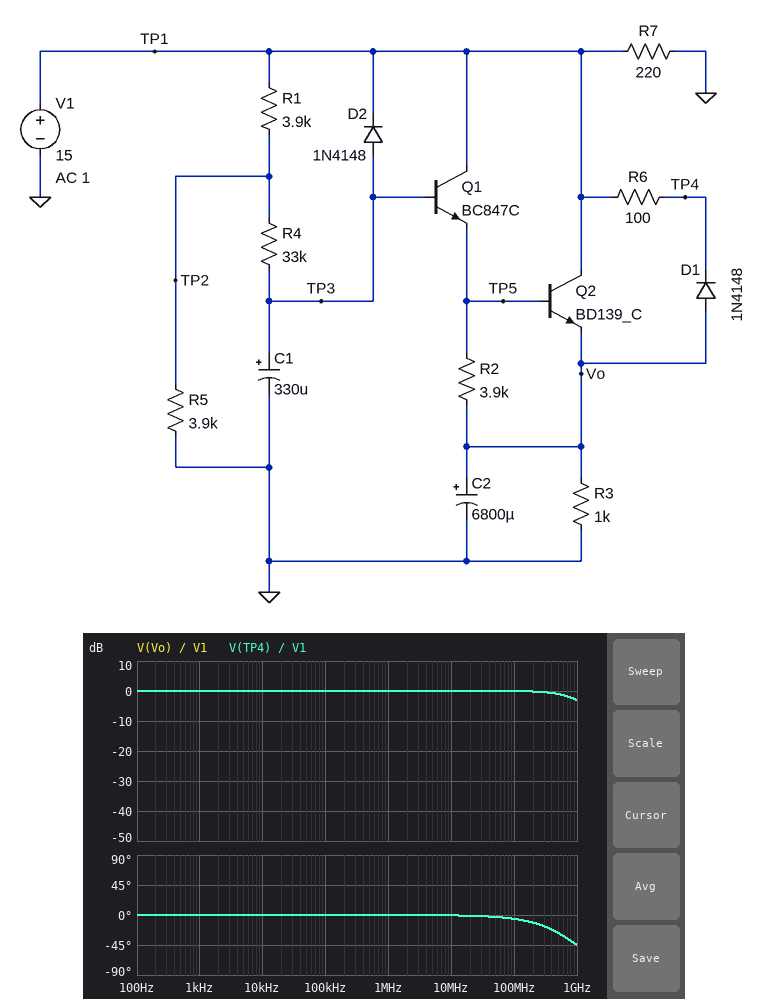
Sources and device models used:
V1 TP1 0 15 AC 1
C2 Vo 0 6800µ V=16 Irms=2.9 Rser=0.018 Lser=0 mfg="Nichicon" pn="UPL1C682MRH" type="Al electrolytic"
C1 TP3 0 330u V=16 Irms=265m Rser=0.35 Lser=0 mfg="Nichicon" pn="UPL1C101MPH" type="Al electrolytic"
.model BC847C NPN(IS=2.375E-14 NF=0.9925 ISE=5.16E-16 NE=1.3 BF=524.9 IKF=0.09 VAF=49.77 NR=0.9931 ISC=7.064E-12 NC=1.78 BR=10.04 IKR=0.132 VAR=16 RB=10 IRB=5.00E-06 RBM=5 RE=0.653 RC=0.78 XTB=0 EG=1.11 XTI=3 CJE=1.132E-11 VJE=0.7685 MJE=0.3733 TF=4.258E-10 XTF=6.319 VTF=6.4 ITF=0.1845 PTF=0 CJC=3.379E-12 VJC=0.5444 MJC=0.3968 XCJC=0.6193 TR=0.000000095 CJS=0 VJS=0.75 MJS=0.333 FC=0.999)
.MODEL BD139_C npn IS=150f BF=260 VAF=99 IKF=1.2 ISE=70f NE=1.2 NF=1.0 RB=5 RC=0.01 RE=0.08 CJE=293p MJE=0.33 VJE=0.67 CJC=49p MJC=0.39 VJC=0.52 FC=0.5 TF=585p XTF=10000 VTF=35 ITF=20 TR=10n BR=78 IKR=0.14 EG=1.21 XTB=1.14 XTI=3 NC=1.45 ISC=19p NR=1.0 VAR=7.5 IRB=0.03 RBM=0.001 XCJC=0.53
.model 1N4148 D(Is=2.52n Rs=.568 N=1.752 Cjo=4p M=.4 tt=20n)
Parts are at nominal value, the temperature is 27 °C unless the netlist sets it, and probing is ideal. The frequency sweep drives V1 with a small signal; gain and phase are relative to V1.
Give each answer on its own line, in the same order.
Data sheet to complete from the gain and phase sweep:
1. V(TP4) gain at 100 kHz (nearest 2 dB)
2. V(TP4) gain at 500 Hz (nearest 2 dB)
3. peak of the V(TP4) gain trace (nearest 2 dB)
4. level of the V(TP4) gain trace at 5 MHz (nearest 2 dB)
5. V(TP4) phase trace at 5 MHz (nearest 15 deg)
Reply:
0 dB
0 dB
0 dB
0 dB
0 deg
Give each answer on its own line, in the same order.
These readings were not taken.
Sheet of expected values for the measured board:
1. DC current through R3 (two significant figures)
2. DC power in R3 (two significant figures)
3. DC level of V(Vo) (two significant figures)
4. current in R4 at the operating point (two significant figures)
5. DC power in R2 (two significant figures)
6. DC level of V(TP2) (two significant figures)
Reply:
6.3 mA
39 mW
6.3 V
420 nA
100 µW
7.5 V
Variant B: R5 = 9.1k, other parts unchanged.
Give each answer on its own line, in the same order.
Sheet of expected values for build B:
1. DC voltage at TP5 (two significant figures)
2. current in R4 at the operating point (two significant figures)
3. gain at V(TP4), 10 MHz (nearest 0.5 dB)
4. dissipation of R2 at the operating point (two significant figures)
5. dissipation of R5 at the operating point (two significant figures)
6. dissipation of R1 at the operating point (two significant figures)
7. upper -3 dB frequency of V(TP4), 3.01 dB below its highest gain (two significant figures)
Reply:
9.9 V
510 nA
0 dB
110 µW
12 mW
5.2 mW
850 MHz
